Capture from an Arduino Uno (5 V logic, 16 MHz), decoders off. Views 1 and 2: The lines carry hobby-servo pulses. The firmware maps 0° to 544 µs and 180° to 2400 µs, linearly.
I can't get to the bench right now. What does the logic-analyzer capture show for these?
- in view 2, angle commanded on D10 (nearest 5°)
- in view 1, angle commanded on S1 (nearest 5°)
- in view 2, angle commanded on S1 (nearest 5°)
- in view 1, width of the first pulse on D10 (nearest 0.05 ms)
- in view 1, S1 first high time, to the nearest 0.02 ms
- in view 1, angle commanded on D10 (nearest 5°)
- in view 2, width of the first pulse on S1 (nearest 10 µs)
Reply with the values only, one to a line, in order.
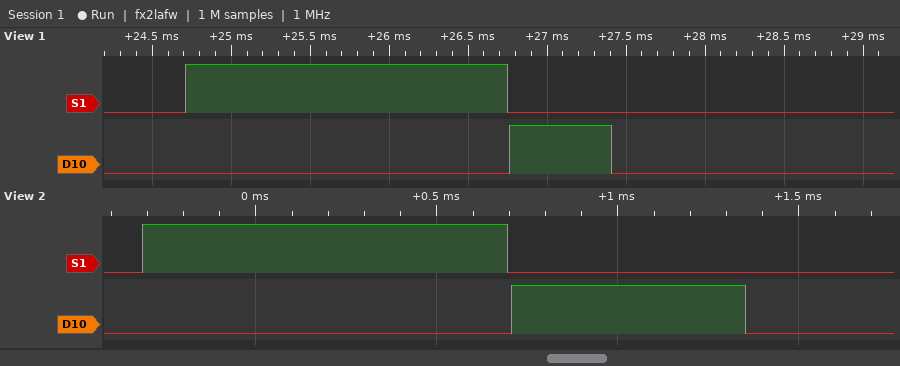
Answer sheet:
10°
145°
45°
0.65 ms
2.04 ms
10°
1010 µs
